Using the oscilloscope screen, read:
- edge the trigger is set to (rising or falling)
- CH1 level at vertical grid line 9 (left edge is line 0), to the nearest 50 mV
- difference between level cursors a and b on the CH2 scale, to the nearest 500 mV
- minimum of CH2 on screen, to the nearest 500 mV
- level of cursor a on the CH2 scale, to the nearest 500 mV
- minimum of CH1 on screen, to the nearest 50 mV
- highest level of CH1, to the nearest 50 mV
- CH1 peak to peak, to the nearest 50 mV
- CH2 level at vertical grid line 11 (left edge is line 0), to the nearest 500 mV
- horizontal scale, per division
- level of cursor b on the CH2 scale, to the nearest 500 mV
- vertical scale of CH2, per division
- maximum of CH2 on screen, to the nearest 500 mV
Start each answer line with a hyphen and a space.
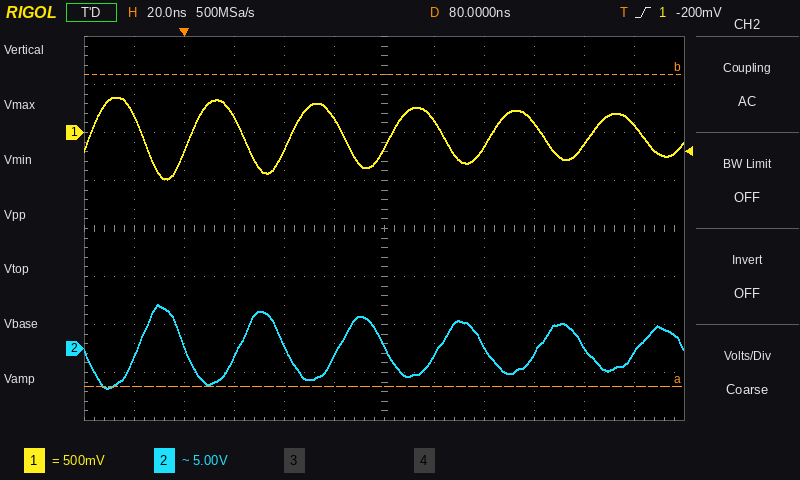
- rising
- 100 mV
- 32.5 V
- -4.0 V
- -4.0 V
- -500 mV
- 350 mV
- 850 mV
- -500 mV
- 20 ns
- 28.5 V
- 5 V
- 4.5 V
